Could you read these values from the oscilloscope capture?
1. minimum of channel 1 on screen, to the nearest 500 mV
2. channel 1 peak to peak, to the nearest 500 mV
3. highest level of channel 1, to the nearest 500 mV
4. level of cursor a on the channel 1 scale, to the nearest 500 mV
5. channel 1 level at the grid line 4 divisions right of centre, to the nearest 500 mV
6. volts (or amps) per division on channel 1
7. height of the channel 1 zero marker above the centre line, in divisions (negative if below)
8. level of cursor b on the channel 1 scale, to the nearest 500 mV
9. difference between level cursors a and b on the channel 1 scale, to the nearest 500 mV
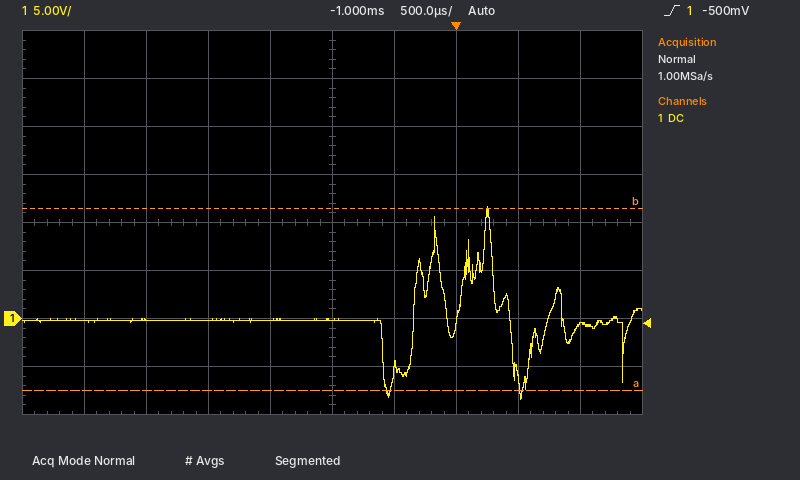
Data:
-8.5 V
20.0 V
11.5 V
-7.5 V
-500 mV
5 V
-2.0 div
11.5 V
19.0 V
